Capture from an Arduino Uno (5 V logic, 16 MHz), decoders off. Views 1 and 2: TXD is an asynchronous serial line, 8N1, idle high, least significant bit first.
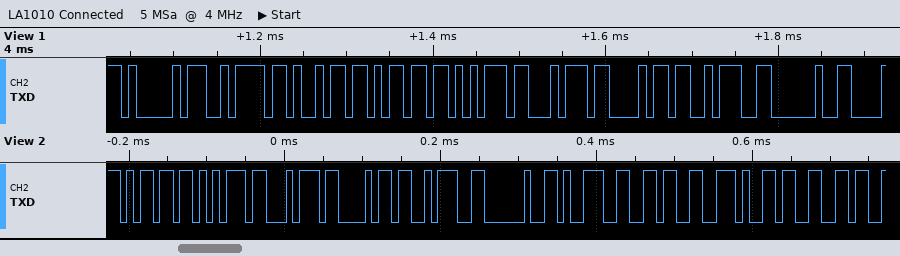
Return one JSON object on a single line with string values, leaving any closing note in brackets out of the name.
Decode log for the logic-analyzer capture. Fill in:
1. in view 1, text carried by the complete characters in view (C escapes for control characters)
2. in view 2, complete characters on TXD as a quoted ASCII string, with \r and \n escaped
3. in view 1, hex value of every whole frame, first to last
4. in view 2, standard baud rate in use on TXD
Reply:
{"in view 1, text carried by the complete characters in view": "\"Azimuth: \"", "in view 2, complete characters on TXD as a quoted ASCII string, with \\r and \\n escaped": "\"muth: 96.3\"", "in view 1, hex value of every whole frame, first to last": "0x41 0x7A 0x69 0x6D 0x75 0x74 0x68 0x3A 0x20", "in view 2, standard baud rate in use on TXD": "115200 baud"}
